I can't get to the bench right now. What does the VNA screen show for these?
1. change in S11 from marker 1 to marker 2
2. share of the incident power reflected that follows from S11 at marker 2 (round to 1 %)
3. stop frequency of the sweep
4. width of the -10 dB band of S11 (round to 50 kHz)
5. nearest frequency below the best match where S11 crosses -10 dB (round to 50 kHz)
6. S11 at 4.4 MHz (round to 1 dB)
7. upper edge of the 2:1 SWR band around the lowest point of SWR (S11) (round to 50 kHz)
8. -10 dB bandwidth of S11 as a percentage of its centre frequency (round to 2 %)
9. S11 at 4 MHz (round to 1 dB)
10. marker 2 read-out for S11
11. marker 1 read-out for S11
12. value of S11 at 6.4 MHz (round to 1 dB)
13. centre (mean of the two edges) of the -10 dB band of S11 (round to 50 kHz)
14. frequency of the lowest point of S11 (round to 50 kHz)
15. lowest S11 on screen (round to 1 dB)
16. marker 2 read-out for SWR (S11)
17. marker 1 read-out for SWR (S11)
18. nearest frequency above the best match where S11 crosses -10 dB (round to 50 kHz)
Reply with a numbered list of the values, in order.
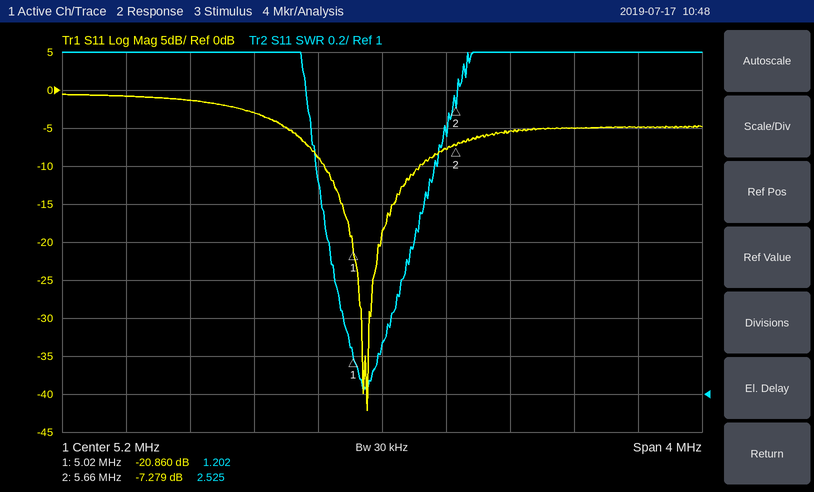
1. 13.581 dB
2. 19 %
3. 7.2 MHz
4. 600 kHz
5. 4.85 MHz
6. -3 dB
7. 5.45 MHz
8. 12 %
9. -1 dB
10. -7.279 dB
11. -20.860 dB
12. -5 dB
13. 5.15 MHz
14. 5.10 MHz
15. -42 dB
16. 2.525
17. 1.202
18. 5.45 MHz
